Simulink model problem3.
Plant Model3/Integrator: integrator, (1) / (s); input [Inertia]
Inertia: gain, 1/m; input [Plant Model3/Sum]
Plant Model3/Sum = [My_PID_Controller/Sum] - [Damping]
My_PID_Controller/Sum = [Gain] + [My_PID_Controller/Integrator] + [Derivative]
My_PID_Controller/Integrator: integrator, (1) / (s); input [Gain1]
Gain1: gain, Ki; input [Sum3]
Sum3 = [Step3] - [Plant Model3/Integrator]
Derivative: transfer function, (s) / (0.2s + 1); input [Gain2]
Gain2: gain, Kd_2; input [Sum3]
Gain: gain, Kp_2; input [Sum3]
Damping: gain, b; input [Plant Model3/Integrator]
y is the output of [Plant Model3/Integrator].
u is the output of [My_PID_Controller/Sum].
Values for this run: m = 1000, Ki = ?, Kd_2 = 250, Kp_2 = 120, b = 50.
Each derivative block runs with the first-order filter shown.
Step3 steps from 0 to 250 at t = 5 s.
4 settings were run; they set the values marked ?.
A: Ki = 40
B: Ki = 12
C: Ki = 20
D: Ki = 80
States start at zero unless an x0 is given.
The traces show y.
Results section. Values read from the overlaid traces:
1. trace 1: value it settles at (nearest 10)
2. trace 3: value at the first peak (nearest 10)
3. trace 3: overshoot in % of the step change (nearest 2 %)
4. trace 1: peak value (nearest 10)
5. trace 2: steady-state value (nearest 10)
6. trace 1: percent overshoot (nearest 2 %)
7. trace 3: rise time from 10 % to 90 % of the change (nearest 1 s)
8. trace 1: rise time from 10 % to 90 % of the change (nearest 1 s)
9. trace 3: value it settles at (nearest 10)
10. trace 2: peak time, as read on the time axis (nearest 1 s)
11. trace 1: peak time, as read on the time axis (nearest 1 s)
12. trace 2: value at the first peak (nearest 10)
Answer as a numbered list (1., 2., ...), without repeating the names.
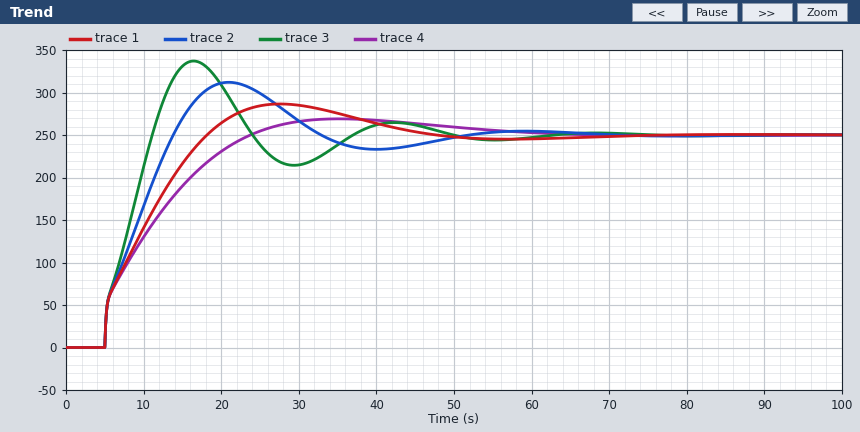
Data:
1. 250
2. 340
3. 34 %
4. 290
5. 250
6. 14 %
7. 5 s
8. 11 s
9. 250
10. 21 s
11. 28 s
12. 310
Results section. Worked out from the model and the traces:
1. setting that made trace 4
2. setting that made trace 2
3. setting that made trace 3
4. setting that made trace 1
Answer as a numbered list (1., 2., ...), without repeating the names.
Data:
1. B
2. A
3. D
4. C
